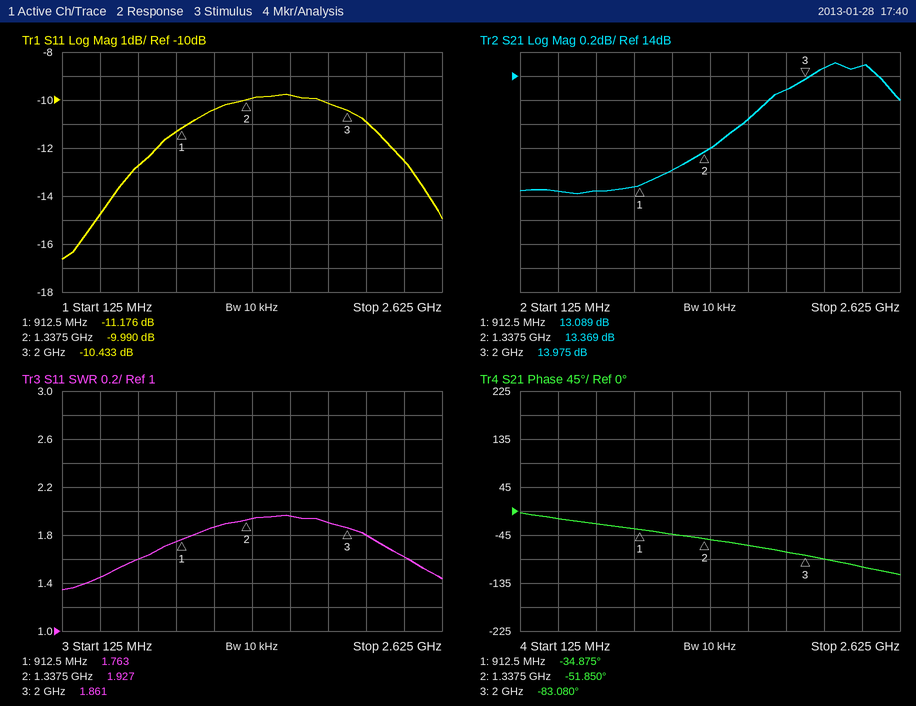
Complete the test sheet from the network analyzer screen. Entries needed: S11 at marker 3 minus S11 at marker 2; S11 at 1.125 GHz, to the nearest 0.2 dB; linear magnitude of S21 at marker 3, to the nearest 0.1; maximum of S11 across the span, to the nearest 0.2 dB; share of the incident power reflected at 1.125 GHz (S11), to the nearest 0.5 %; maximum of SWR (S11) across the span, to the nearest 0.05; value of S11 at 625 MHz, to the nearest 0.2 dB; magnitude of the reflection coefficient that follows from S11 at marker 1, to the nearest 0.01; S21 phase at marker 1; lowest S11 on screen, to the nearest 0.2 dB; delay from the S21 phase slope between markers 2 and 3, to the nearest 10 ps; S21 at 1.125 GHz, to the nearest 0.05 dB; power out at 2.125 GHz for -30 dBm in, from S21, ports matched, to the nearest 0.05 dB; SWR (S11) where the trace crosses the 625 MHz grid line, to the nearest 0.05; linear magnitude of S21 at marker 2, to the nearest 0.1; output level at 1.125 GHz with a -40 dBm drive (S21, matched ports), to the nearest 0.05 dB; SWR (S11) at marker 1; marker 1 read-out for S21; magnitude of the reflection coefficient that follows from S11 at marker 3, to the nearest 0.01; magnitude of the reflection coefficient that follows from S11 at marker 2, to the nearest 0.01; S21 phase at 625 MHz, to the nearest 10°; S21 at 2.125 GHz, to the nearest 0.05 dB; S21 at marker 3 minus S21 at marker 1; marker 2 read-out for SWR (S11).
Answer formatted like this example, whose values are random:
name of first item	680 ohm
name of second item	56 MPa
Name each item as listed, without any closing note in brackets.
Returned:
S11 at marker 3 minus S11 at marker 2	-0.443 dB
S11 at 1.125 GHz, to the nearest 0.2 dB	-10.4 dB
linear magnitude of S21 at marker 3, to the nearest 0.1	5.0
maximum of S11 across the span, to the nearest 0.2 dB	-9.8 dB
share of the incident power reflected at 1.125 GHz (S11), to the nearest 0.5 %	9.0 %
maximum of SWR (S11) across the span, to the nearest 0.05	1.95
value of S11 at 625 MHz, to the nearest 0.2 dB	-12.8 dB
magnitude of the reflection coefficient that follows from S11 at marker 1, to the nearest 0.01	0.28
S21 phase at marker 1	-34.875°
lowest S11 on screen, to the nearest 0.2 dB	-16.6 dB
delay from the S21 phase slope between markers 2 and 3, to the nearest 10 ps	130 ps
S21 at 1.125 GHz, to the nearest 0.05 dB	13.20 dB
power out at 2.125 GHz for -30 dBm in, from S21, ports matched, to the nearest 0.05 dB	-15.95 dBm
SWR (S11) where the trace crosses the 625 MHz grid line, to the nearest 0.05	1.60
linear magnitude of S21 at marker 2, to the nearest 0.1	4.7
output level at 1.125 GHz with a -40 dBm drive (S21, matched ports), to the nearest 0.05 dB	-26.80 dBm
SWR (S11) at marker 1	1.763
marker 1 read-out for S21	13.089 dB
magnitude of the reflection coefficient that follows from S11 at marker 3, to the nearest 0.01	0.30
magnitude of the reflection coefficient that follows from S11 at marker 2, to the nearest 0.01	0.32
S21 phase at 625 MHz, to the nearest 10°	-20°
S21 at 2.125 GHz, to the nearest 0.05 dB	14.05 dB
S21 at marker 3 minus S21 at marker 1	0.886 dB
marker 2 read-out for SWR	1.927
